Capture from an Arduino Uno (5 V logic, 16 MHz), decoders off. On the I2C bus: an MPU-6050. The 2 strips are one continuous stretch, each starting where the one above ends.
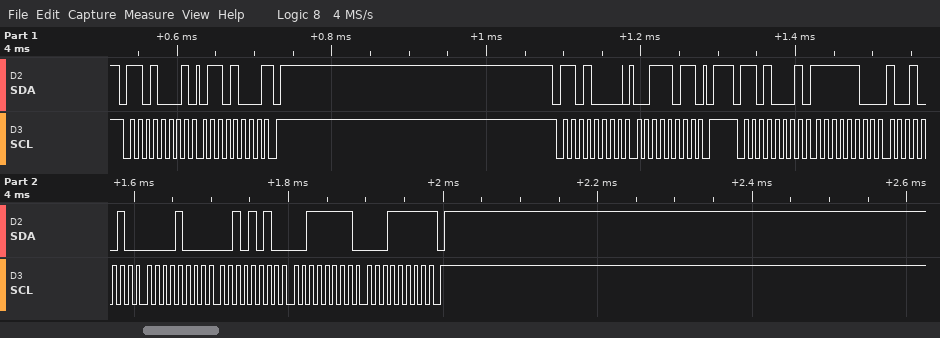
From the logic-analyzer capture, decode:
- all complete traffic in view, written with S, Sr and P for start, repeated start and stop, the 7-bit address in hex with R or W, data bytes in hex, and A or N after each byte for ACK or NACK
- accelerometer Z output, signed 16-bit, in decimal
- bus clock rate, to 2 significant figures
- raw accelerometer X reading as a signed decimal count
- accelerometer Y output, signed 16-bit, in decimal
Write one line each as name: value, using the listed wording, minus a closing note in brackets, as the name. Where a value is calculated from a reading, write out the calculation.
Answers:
all complete traffic in view, written with S, Sr and P for start, repeated start and stop, the 7-bit address in hex with R or W, data bytes in hex, and A or N after each byte for ACK or NACK: S 68R A 68 N P S 68W A 3B A P S 68R A FC A 92 A 08 A 2A A 3F A 1F N P
accelerometer Z output, signed 16-bit, in decimal: 0x3F1F = 16159
bus clock rate, to 2 significant figures: 100 kHz
raw accelerometer X reading as a signed decimal count: 0xFC92 = -878
accelerometer Y output, signed 16-bit, in decimal: 0x082A = 2090
